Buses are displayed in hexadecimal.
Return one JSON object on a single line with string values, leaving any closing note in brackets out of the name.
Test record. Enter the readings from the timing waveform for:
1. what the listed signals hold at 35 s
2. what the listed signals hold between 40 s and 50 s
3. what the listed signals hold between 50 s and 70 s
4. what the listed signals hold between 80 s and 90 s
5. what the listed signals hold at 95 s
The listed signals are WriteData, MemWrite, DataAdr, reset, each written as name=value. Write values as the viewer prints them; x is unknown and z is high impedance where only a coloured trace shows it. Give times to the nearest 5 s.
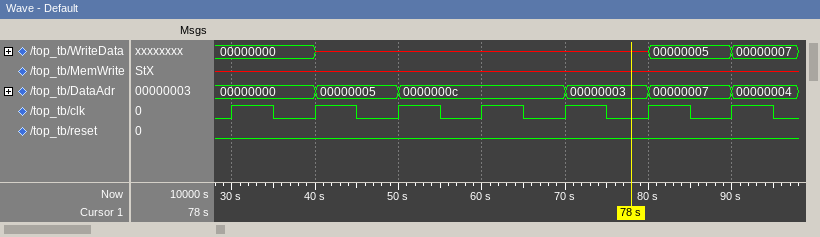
{"what the listed signals hold at 35 s": "WriteData=00000000, MemWrite=x, DataAdr=00000000, reset=0", "what the listed signals hold between 40 s and 50 s": "WriteData=x, MemWrite=x, DataAdr=00000005, reset=0", "what the listed signals hold between 50 s and 70 s": "WriteData=x, MemWrite=x, DataAdr=0000000c, reset=0", "what the listed signals hold between 80 s and 90 s": "WriteData=00000005, MemWrite=x, DataAdr=00000007, reset=0", "what the listed signals hold at 95 s": "WriteData=00000007, MemWrite=x, DataAdr=00000004, reset=0"}
